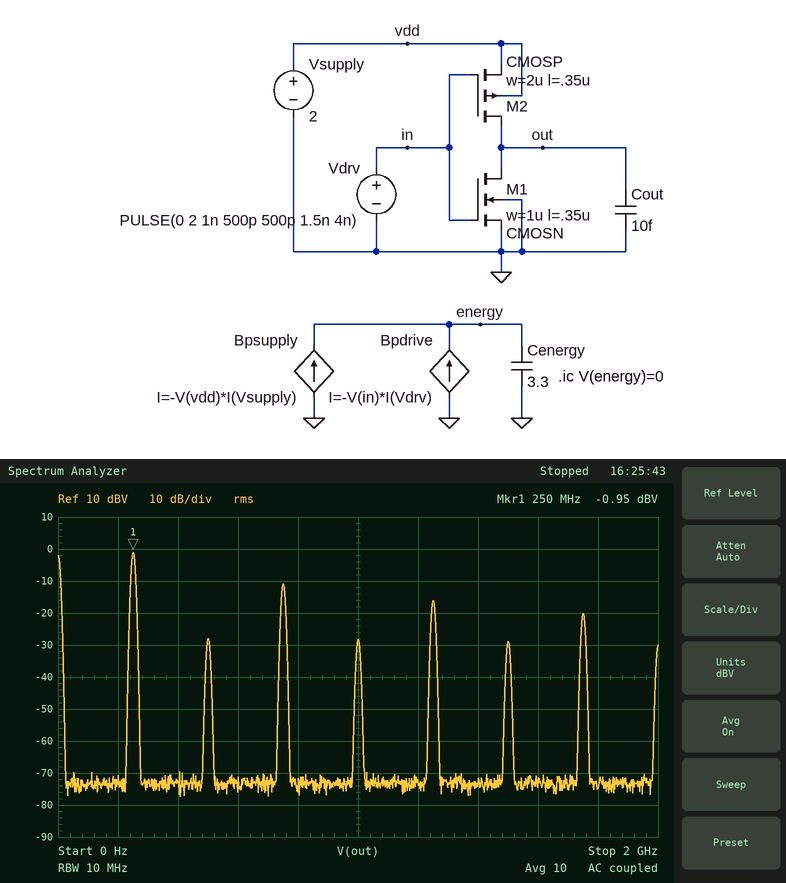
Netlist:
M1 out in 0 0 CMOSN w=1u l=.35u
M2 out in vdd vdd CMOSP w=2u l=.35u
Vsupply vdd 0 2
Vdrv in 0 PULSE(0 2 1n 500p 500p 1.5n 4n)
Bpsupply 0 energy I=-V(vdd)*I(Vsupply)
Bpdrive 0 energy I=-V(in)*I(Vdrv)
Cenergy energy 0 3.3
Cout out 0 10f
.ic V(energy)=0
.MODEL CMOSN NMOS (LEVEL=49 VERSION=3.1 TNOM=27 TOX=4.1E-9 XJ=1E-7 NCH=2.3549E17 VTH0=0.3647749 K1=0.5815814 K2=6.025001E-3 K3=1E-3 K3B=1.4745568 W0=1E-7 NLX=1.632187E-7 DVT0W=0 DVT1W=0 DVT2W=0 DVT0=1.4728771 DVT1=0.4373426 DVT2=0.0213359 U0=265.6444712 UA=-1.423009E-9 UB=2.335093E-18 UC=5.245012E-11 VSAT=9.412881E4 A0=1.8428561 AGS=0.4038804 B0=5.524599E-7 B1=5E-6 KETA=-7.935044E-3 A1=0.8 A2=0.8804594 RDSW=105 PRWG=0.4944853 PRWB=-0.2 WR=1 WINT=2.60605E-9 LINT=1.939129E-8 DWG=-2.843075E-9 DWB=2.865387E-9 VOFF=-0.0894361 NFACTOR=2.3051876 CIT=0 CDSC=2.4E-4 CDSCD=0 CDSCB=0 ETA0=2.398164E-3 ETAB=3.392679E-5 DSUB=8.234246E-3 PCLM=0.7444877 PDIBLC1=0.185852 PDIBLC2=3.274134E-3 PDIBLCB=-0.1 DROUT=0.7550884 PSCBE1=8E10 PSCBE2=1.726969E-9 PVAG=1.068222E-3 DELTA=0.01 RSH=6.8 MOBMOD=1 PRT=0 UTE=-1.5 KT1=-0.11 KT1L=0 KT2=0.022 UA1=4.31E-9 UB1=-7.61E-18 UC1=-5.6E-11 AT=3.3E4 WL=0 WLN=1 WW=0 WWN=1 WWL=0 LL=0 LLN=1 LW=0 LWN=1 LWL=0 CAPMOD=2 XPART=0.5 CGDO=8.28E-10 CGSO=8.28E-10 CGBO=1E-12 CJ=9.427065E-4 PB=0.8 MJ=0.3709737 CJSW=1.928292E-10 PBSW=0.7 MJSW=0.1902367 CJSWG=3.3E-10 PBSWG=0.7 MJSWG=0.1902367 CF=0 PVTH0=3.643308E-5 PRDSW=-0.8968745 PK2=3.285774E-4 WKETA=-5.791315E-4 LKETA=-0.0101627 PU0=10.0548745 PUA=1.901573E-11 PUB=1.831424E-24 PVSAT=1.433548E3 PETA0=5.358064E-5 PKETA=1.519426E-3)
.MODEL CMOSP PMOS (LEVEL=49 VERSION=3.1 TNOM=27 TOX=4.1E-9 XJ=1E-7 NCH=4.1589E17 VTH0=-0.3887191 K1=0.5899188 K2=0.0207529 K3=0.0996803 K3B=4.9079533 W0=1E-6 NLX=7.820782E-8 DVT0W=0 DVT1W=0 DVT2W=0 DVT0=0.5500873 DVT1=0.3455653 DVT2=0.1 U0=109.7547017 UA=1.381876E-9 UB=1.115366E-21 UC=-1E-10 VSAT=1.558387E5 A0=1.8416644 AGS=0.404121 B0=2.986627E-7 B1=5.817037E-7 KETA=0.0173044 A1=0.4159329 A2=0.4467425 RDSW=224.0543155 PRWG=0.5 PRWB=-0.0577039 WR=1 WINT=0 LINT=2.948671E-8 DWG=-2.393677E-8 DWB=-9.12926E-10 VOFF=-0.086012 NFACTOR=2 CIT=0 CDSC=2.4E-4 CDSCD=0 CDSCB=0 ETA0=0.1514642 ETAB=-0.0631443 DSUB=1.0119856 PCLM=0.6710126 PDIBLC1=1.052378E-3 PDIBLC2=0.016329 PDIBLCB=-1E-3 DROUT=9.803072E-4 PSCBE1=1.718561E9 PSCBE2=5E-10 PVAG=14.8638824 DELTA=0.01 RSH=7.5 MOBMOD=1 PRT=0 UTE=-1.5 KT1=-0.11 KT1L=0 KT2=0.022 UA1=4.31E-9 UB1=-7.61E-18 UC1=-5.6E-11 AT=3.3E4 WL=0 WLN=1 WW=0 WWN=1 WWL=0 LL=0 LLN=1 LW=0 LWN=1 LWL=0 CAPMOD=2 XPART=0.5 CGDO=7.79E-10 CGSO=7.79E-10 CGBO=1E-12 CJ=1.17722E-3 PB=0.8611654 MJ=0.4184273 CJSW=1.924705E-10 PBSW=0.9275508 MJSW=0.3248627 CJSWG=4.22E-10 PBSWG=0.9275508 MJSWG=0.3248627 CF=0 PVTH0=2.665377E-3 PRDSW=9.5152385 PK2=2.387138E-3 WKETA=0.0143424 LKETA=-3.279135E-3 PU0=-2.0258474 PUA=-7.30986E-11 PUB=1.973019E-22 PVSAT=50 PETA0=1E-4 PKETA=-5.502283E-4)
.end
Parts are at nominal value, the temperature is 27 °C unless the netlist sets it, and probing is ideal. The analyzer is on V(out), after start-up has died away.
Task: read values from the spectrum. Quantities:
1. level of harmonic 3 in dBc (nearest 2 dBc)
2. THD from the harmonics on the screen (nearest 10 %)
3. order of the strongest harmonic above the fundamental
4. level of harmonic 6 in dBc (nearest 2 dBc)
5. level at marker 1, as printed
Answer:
-10 dBc
40 %
3
-28 dBc
-0.95 dBV
